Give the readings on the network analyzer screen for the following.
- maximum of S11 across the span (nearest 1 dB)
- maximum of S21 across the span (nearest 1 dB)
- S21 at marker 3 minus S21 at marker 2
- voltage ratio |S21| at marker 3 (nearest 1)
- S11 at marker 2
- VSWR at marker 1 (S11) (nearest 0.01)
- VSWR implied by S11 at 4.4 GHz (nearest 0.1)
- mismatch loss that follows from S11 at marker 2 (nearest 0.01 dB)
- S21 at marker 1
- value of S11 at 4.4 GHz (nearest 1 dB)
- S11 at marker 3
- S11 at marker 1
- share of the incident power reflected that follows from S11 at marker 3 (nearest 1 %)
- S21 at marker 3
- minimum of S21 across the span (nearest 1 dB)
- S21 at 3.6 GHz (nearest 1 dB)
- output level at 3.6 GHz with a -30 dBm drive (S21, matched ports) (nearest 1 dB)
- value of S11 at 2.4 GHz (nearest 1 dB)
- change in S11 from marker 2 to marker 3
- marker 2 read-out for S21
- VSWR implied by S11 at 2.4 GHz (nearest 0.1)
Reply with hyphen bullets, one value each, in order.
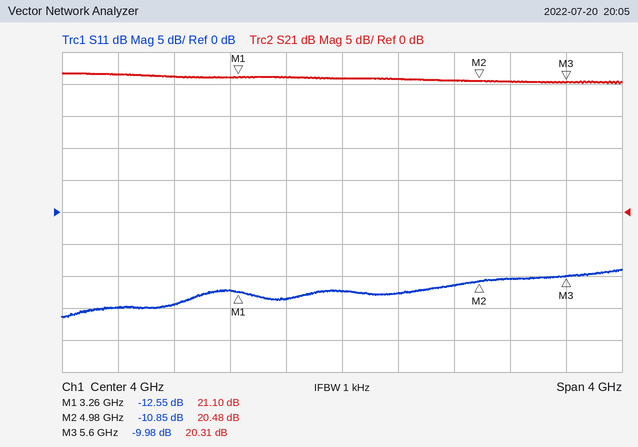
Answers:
- -9 dB
- 22 dB
- -0.17 dB
- 10
- -10.85 dB
- 1.62
- 1.6
- 0.37 dB
- 21.10 dB
- -13 dB
- -9.98 dB
- -12.55 dB
- 10 %
- 20.31 dB
- 20 dB
- 21 dB
- -9 dBm
- -15 dB
- 0.87 dB
- 20.48 dB
- 1.4
